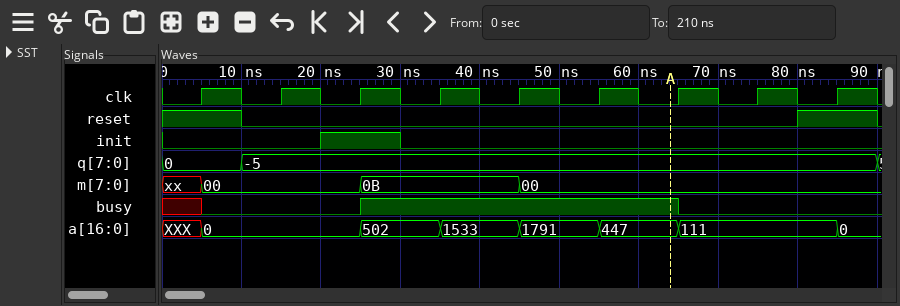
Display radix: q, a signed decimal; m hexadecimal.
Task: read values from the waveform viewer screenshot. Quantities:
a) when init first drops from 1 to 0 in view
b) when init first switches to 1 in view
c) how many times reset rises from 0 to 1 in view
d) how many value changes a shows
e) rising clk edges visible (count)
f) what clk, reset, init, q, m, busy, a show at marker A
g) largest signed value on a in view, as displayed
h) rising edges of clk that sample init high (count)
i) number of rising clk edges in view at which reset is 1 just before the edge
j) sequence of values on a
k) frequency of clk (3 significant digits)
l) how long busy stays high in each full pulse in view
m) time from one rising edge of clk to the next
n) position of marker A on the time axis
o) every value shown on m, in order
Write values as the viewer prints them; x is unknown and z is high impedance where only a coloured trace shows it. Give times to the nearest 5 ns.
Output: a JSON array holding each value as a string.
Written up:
["30 ns", "20 ns", "1", "7", "9", "clk=0, reset=0, init=0, q=-5, m=00, busy=1, a=447", "1791", "1", "2", "XXX, 0, 502, 1533, 1791, 447, 111, 0", "100 MHz", "40 ns", "10 ns", "65 ns", "xx, 00, 0B, 00"]
